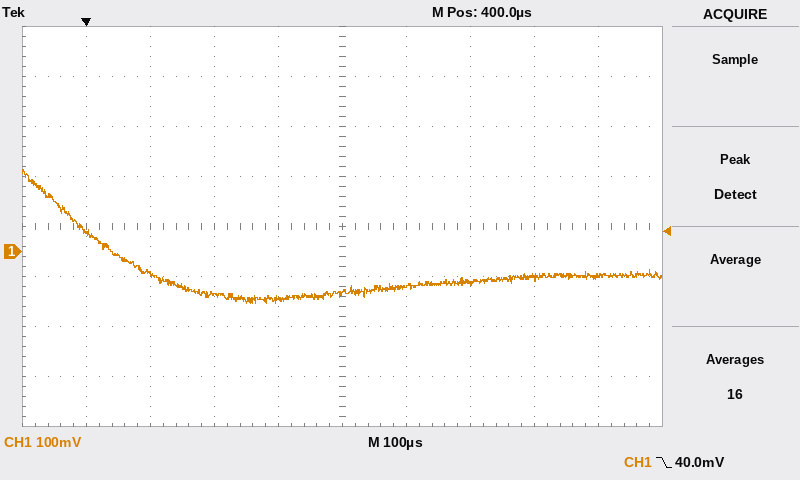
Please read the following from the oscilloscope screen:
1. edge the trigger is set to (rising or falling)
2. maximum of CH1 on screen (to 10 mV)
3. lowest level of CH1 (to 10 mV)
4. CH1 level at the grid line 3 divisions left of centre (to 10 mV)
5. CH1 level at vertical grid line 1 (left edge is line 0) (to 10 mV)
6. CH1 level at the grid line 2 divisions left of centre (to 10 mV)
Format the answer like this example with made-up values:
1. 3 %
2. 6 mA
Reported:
1. falling
2. 160 mV
3. -100 mV
4. -40 mV
5. 40 mV
6. -80 mV
